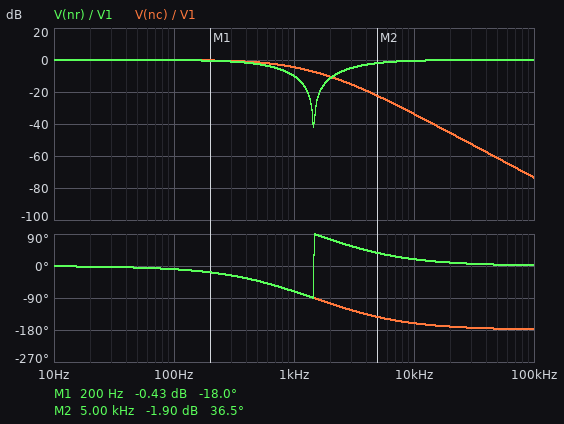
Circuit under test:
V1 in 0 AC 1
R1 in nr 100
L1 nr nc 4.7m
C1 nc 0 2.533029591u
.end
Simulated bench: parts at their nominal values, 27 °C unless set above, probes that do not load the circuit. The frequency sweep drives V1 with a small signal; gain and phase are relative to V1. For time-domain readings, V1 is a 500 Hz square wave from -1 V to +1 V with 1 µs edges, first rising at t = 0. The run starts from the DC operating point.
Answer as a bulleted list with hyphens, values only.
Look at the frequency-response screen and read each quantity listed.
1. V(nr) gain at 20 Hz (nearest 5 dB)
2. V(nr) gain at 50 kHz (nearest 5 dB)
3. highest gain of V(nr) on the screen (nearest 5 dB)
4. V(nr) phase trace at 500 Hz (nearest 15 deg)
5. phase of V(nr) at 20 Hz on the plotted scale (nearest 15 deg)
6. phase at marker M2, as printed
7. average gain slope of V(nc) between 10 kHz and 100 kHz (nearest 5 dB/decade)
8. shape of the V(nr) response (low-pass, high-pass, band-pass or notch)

- 0 dB
- 0 dB
- 0 dB
- -45 deg
- 0 deg
- 36.5 deg
- -40 dB/decade
- notch
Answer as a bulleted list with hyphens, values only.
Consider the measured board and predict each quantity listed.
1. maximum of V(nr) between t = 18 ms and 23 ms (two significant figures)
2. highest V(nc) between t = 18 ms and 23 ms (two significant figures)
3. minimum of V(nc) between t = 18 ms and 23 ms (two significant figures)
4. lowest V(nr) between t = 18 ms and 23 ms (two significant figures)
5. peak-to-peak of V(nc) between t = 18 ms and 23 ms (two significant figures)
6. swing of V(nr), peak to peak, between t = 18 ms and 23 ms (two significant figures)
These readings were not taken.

- 1.0 V
- 980 mV
- -980 mV
- -1.0 V
- 2.0 V
- 2.0 V
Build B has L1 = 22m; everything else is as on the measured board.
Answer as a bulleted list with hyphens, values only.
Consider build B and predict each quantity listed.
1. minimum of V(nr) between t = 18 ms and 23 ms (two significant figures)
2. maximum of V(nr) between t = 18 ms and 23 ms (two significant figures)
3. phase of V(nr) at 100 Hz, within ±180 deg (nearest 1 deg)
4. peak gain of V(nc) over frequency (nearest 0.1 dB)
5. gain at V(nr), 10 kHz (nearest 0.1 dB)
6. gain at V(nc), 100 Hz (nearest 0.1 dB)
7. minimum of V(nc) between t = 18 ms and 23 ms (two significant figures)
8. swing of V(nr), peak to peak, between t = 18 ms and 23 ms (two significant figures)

- -1.1 V
- 1.1 V
- -9 deg
- 0.9 dB
- 0 dB
- 0.1 dB
- -1.3 V
- 2.3 V
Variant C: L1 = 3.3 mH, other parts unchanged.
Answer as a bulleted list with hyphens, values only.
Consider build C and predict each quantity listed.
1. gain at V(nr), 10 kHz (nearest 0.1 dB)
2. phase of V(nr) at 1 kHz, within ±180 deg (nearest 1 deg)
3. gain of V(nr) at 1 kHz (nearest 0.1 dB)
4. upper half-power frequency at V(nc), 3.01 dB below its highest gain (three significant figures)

- -1.0 dB
- -67 deg
- -8.2 dB
- 720 Hz
